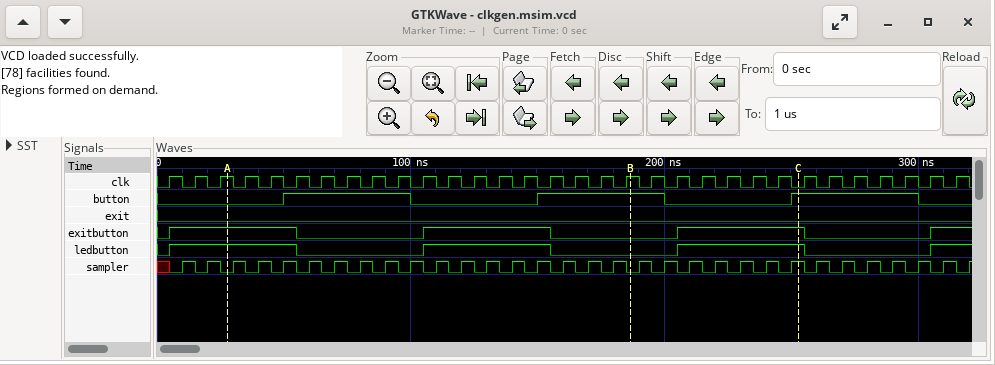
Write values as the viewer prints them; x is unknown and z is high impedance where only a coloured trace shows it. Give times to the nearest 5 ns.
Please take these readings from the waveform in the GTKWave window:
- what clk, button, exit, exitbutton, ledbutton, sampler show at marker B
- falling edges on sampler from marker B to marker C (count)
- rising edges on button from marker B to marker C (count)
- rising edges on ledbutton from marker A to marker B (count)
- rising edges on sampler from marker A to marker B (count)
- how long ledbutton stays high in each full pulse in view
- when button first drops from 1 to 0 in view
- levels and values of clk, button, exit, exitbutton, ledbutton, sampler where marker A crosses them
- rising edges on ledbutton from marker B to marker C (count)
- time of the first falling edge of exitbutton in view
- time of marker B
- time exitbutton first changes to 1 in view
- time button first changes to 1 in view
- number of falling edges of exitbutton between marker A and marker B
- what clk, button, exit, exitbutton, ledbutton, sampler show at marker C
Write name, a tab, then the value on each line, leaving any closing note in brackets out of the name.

what clk, button, exit, exitbutton, ledbutton, sampler show at marker B	clk=1, button=1, exit=0, exitbutton=0, ledbutton=0, sampler=0
falling edges on sampler from marker B to marker C	6
rising edges on button from marker B to marker C	1
rising edges on ledbutton from marker A to marker B	1
rising edges on sampler from marker A to marker B	16
how long ledbutton stays high in each full pulse in view	50 ns, 50 ns, 50 ns
when button first drops from 1 to 0 in view	100 ns
levels and values of clk, button, exit, exitbutton, ledbutton, sampler where marker A crosses them	clk=1, button=0, exit=0, exitbutton=1, ledbutton=1, sampler=0
rising edges on ledbutton from marker B to marker C	1
time of the first falling edge of exitbutton in view	55 ns
time of marker B	185 ns
time exitbutton first changes to 1 in view	5 ns
time button first changes to 1 in view	50 ns
number of falling edges of exitbutton between marker A and marker B	2
what clk, button, exit, exitbutton, ledbutton, sampler show at marker C	clk=0, button=1, exit=0, exitbutton=1, ledbutton=1, sampler=1
